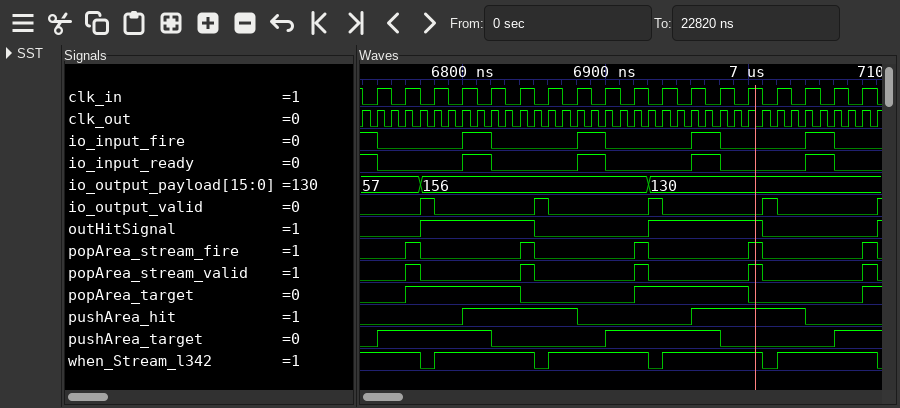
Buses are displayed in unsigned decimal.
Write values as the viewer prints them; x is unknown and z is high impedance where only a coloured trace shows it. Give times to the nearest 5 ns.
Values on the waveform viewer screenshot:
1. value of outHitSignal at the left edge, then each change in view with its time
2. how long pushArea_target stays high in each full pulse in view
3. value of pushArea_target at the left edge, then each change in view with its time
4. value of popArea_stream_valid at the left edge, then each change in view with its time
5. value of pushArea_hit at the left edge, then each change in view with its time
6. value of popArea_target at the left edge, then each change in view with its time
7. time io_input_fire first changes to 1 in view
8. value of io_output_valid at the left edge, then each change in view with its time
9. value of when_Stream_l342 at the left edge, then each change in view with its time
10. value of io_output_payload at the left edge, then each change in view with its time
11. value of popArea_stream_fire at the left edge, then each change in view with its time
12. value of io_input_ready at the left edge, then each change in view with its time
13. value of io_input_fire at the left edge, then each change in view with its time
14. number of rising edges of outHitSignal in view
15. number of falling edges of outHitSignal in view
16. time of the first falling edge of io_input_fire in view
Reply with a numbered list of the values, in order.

1. 0, 1 at 6770 ns, 0 at 6850 ns, 1 at 6930 ns, 0 at 7010 ns, 1 at 7090 ns
2. 80 ns, 80 ns
3. 0, 1 at 6740 ns, 0 at 6820 ns, 1 at 6900 ns, 0 at 6980 ns, 1 at 7060 ns
4. 0, 1 at 6760 ns, 0 at 6770 ns, 1 at 6840 ns, 0 at 6850 ns, 1 at 6920 ns, 0 at 6930 ns, 1 at 7000 ns, 0 at 7010 ns, 1 at 7080 ns, 0 at 7090 ns
5. 0, 1 at 6800 ns, 0 at 6880 ns, 1 at 6960 ns, 0 at 7040 ns
6. 0, 1 at 6760 ns, 0 at 6840 ns, 1 at 6920 ns, 0 at 7000 ns, 1 at 7080 ns
7. 6800 ns
8. 0, 1 at 6770 ns, 0 at 6780 ns, 1 at 6850 ns, 0 at 6860 ns, 1 at 6930 ns, 0 at 6940 ns, 1 at 7010 ns, 0 at 7020 ns, 1 at 7090 ns
9. 1, 0 at 6770 ns, 1 at 6780 ns, 0 at 6850 ns, 1 at 6860 ns, 0 at 6930 ns, 1 at 6940 ns, 0 at 7010 ns, 1 at 7020 ns, 0 at 7090 ns
10. 57, 156 at 6770 ns, 130 at 6930 ns
11. 0, 1 at 6760 ns, 0 at 6770 ns, 1 at 6840 ns, 0 at 6850 ns, 1 at 6920 ns, 0 at 6930 ns, 1 at 7000 ns, 0 at 7010 ns, 1 at 7080 ns, 0 at 7090 ns
12. 1, 0 at 6740 ns, 1 at 6800 ns, 0 at 6820 ns, 1 at 6880 ns, 0 at 6900 ns, 1 at 6960 ns, 0 at 6980 ns, 1 at 7040 ns, 0 at 7060 ns
13. 1, 0 at 6740 ns, 1 at 6800 ns, 0 at 6820 ns, 1 at 6880 ns, 0 at 6900 ns, 1 at 6960 ns, 0 at 6980 ns, 1 at 7040 ns, 0 at 7060 ns
14. 3
15. 2
16. 6740 ns
